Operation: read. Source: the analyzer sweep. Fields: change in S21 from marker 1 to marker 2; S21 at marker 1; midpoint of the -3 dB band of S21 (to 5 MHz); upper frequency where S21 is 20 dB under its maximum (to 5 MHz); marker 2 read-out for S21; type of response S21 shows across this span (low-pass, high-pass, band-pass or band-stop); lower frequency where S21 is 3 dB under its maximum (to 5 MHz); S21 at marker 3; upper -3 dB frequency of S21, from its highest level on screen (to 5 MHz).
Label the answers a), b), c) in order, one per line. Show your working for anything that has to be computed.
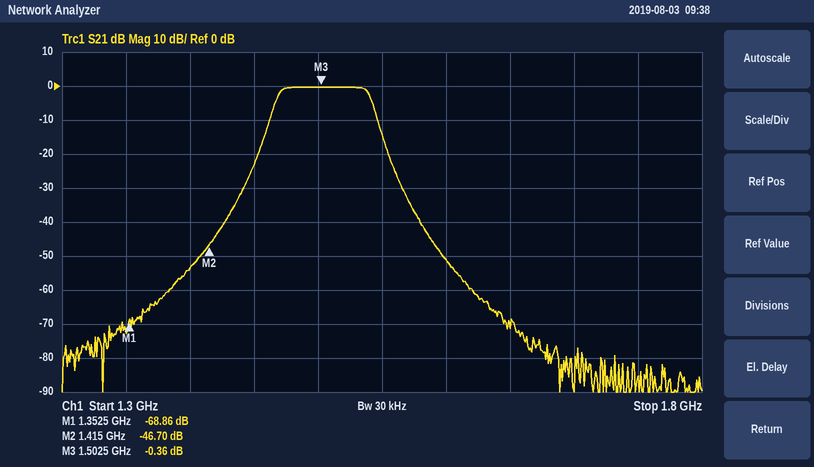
a) -46.7 − (-68.86) = 22.16 dB
b) -68.86 dB
c) 1.505 GHz
d) 1.555 GHz
e) -46.70 dB
f) band-pass
g) 1.470 GHz
h) -0.36 dB
i) 1.540 GHz
